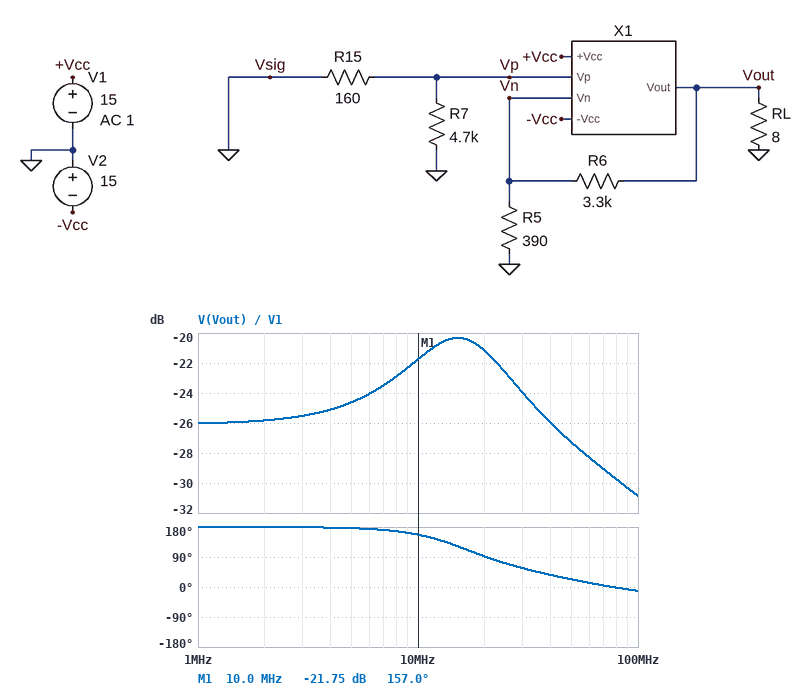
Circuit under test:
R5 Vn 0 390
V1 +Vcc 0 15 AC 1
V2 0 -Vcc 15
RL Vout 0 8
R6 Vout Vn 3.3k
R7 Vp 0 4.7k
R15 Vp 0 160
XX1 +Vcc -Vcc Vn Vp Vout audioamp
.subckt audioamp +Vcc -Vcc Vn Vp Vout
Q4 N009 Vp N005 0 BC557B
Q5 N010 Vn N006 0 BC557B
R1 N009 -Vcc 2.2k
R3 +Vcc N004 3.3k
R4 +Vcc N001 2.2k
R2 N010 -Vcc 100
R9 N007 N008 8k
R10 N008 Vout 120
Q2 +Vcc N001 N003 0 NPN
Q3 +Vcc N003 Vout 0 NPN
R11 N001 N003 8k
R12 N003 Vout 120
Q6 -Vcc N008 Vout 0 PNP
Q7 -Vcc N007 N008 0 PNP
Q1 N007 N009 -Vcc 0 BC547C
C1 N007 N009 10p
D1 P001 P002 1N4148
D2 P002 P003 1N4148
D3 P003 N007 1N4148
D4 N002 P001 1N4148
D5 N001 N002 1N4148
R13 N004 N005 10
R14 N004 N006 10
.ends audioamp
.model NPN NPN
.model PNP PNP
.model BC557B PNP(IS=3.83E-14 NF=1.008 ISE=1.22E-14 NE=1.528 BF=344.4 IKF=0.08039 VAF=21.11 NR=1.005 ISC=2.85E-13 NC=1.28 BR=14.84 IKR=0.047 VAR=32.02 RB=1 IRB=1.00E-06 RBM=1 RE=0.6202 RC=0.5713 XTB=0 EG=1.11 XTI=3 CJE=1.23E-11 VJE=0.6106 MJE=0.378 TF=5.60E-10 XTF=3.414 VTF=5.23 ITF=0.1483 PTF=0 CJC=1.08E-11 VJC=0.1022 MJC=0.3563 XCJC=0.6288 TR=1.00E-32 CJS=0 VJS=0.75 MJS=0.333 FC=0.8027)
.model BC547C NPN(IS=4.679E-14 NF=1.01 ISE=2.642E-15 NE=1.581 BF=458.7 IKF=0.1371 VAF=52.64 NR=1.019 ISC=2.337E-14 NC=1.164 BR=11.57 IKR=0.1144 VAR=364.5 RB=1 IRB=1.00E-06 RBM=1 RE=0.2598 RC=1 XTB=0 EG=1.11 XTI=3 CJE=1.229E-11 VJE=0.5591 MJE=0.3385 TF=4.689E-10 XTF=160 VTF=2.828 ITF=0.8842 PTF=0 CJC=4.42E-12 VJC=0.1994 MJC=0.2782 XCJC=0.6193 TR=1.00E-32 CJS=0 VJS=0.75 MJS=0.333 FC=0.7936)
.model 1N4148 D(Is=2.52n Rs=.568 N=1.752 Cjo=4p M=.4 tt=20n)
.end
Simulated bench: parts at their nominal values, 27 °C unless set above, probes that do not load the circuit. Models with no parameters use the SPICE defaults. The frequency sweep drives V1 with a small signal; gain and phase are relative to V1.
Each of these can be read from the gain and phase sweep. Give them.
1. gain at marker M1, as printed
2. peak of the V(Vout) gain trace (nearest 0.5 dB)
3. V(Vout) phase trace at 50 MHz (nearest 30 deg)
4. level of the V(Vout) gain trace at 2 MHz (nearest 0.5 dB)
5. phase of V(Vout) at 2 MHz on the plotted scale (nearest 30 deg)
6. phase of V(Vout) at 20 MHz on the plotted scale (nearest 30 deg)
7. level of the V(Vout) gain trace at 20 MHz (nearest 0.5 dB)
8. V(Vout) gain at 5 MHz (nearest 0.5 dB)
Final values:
-21.75 dB
-20.5 dB
30 deg
-26.0 dB
180 deg
90 deg
-21.0 dB
-24.5 dB
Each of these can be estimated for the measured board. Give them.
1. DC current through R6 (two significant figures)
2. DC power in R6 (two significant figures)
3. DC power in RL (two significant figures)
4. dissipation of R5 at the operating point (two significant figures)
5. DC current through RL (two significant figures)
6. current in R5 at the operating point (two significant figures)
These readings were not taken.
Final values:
280 µA
260 µW
130 mW
29 µW
130 mA
270 µA
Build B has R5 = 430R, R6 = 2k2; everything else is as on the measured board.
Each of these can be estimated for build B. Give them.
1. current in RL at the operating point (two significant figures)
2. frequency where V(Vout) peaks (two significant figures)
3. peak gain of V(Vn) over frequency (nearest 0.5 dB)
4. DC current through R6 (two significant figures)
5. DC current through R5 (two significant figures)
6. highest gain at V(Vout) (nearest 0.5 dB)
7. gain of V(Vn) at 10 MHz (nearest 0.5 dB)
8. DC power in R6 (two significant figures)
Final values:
84 mA
19 MHz
-31.5 dB
260 µA
250 µA
-19.5 dB
-39.5 dB
140 µW
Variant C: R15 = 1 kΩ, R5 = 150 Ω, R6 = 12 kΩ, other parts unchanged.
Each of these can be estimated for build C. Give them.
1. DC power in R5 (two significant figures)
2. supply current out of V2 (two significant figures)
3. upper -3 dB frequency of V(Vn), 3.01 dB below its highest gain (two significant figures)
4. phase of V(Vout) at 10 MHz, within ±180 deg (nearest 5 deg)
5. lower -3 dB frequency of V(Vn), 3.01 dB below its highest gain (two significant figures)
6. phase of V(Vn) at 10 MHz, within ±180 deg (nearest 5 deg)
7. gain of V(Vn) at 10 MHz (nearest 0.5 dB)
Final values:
73 µW
1.1 A
560 MHz
40 deg
94 MHz
75 deg
-50.5 dB
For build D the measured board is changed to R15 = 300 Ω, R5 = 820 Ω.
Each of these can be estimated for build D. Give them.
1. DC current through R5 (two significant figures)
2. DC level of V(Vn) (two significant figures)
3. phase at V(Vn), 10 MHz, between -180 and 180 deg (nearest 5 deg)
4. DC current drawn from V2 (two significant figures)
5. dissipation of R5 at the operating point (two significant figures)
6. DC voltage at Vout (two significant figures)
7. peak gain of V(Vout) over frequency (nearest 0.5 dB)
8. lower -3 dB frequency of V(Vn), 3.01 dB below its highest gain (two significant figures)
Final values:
130 µA
-110 mV
145 deg
92 mA
14 µW
-560 mV
-14.0 dB
13 MHz
